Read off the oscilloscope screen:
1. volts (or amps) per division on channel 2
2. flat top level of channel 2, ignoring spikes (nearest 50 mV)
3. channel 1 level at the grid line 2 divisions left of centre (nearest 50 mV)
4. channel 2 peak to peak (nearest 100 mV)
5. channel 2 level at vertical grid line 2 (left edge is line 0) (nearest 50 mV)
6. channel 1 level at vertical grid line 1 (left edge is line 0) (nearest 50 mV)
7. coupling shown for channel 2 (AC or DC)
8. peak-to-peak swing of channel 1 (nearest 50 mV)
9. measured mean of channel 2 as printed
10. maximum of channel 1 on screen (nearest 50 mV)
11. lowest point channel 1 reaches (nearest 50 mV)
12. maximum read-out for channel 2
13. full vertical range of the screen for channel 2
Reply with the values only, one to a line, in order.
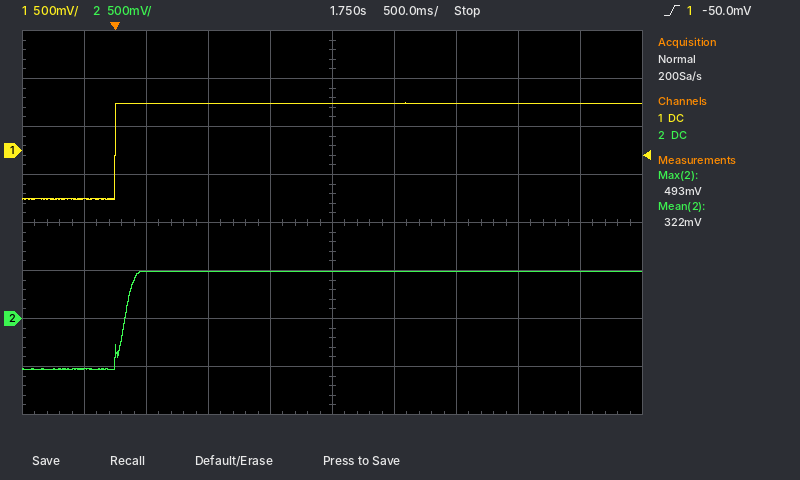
500 mV
500 mV
500 mV
1.00 V
500 mV
-500 mV
DC
1.00 V
322 mV
500 mV
-500 mV
493 mV
4 V
